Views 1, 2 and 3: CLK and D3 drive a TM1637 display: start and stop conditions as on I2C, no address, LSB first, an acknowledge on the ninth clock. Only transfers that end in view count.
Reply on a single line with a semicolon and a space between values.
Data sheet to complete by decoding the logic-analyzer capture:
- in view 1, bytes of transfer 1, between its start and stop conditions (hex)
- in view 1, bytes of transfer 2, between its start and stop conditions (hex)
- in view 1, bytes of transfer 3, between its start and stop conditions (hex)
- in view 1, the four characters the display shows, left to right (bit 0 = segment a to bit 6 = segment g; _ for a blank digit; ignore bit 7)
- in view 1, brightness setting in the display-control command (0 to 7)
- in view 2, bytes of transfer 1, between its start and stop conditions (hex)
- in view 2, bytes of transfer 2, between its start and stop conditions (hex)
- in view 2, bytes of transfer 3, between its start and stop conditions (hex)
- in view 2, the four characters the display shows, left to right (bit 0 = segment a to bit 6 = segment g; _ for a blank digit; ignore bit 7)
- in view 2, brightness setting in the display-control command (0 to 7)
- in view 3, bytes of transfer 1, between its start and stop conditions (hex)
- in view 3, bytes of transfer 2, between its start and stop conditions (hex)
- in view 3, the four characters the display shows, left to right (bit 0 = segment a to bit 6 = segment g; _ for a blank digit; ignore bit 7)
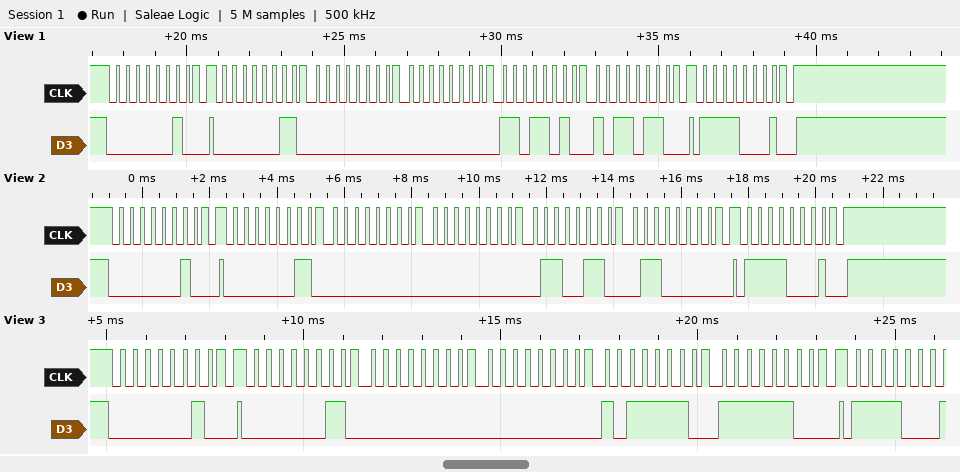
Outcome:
40; C0 00 00 5B 6D; 8F; __25; 7; 40; C0 00 00 66 06; 8F; __41; 7; 40; C0 00 00 7D 3F; __60
